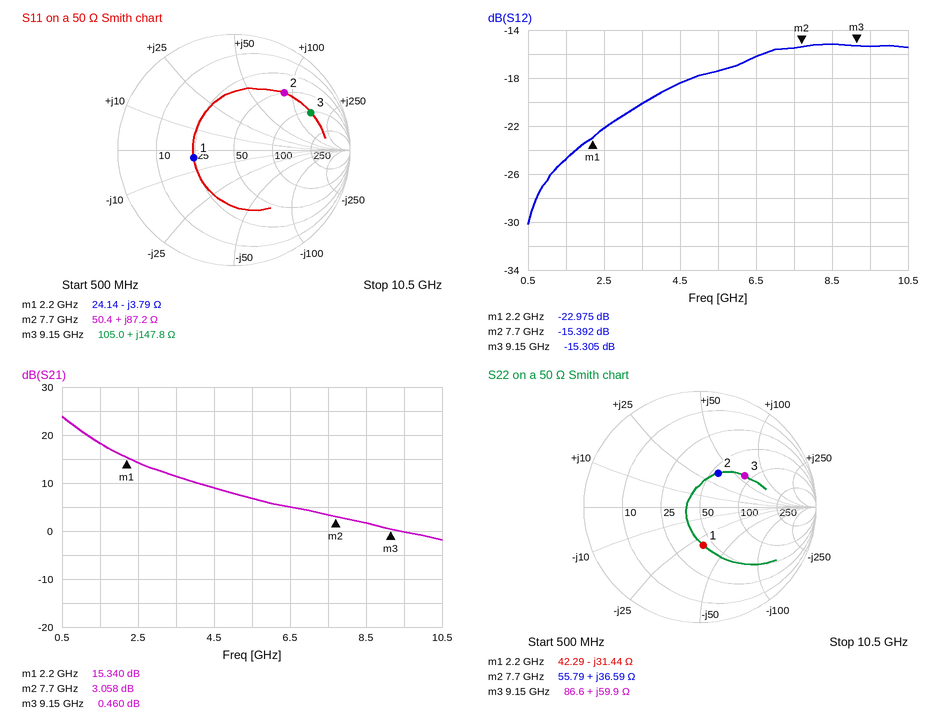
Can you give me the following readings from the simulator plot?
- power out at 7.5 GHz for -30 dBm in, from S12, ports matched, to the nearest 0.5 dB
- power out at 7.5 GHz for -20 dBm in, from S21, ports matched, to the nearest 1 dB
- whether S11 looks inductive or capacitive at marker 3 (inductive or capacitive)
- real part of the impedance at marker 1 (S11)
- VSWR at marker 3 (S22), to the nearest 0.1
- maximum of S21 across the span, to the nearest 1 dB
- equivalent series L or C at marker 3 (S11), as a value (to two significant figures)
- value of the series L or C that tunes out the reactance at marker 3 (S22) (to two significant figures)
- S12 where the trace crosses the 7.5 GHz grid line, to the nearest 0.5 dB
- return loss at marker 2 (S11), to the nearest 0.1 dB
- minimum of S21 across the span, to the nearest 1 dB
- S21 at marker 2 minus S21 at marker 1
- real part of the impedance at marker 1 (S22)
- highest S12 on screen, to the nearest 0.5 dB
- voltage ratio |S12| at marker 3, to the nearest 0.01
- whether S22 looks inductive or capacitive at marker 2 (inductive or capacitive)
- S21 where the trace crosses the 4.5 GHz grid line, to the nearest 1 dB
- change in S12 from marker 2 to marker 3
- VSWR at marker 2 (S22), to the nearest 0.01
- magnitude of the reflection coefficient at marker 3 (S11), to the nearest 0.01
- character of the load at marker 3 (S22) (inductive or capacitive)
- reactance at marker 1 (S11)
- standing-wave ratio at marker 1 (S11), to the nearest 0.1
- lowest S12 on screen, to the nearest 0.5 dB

-45.5 dBm
-17 dBm
inductive
24.14 Ω
2.8
24 dB
2.6 nH
290 fF
-15.5 dB
3.7 dB
-2 dB
-12.282 dB
42.29 Ω
-15.0 dB
0.17
inductive
9 dB
0.087 dB
1.99
0.74
inductive
-3.79 Ω
2.1
-30.0 dB
